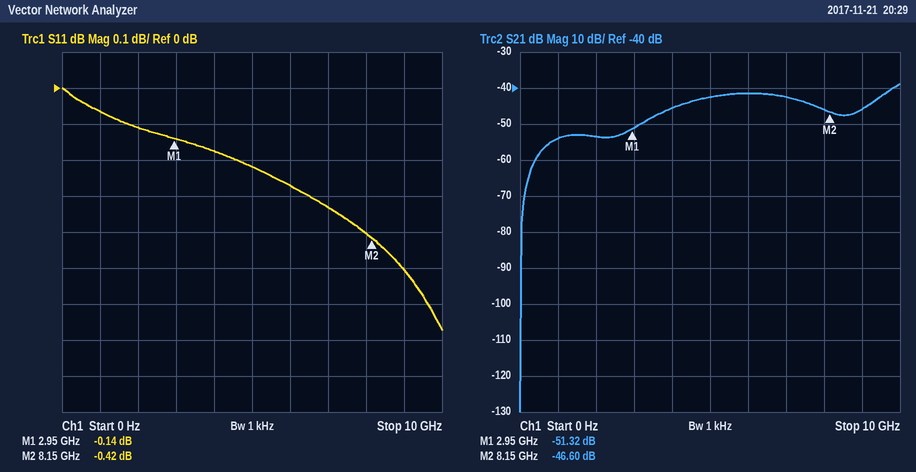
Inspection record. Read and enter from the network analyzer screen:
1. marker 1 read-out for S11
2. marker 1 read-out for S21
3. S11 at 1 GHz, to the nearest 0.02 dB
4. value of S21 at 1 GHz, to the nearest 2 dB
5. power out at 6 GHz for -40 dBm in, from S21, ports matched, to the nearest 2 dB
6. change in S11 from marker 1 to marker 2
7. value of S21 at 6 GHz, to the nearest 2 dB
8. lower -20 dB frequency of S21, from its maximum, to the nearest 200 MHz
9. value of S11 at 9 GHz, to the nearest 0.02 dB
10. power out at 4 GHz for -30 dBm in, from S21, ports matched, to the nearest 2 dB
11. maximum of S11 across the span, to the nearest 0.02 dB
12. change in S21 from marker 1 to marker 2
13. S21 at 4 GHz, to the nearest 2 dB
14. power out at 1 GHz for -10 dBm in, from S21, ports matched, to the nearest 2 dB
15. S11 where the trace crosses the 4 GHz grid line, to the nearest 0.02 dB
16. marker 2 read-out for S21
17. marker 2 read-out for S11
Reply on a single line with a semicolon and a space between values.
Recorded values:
-0.14 dB; -51.32 dB; -0.06 dB; -54 dB; -82 dBm; -0.28 dB; -42 dB; 400 MHz; -0.50 dB; -76 dBm; 0.00 dB; 4.72 dB; -46 dB; -64 dBm; -0.18 dB; -46.60 dB; -0.42 dB
